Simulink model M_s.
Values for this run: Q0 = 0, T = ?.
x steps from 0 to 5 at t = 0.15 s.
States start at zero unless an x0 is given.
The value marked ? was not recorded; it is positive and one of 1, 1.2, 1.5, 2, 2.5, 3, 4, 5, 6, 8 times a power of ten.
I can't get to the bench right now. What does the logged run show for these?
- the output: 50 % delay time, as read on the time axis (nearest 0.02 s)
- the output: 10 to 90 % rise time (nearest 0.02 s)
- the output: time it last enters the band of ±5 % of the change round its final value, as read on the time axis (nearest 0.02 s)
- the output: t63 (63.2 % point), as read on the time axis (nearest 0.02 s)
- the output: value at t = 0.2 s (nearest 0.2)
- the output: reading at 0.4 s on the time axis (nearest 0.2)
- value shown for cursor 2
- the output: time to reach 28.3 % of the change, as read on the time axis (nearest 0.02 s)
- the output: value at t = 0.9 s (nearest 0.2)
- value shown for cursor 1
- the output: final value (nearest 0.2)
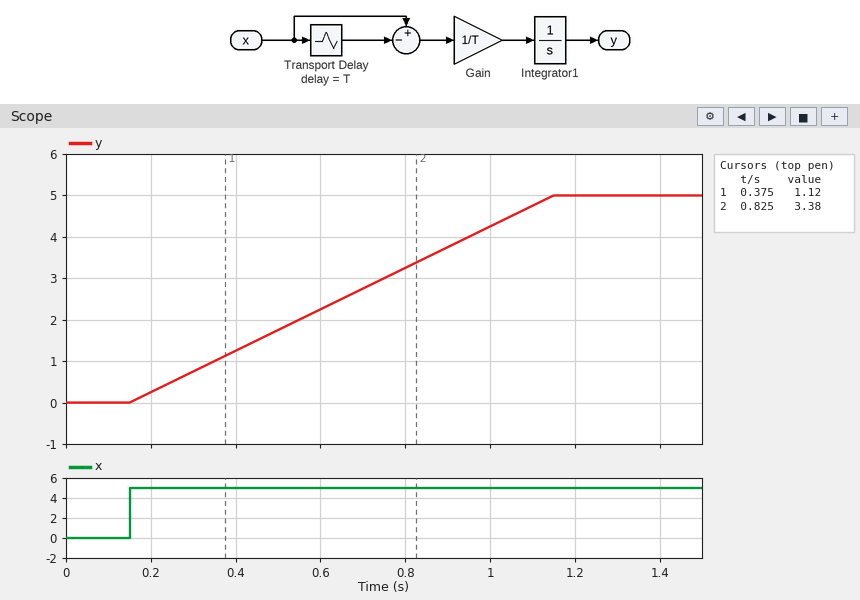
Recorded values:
0.64 s
0.80 s
1.10 s
0.78 s
0.2
1.2
3.38
0.44 s
3.8
1.12
5.0
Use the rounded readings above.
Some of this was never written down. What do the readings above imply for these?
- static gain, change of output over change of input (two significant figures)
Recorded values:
1.0
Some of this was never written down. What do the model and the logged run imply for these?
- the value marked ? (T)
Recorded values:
1
